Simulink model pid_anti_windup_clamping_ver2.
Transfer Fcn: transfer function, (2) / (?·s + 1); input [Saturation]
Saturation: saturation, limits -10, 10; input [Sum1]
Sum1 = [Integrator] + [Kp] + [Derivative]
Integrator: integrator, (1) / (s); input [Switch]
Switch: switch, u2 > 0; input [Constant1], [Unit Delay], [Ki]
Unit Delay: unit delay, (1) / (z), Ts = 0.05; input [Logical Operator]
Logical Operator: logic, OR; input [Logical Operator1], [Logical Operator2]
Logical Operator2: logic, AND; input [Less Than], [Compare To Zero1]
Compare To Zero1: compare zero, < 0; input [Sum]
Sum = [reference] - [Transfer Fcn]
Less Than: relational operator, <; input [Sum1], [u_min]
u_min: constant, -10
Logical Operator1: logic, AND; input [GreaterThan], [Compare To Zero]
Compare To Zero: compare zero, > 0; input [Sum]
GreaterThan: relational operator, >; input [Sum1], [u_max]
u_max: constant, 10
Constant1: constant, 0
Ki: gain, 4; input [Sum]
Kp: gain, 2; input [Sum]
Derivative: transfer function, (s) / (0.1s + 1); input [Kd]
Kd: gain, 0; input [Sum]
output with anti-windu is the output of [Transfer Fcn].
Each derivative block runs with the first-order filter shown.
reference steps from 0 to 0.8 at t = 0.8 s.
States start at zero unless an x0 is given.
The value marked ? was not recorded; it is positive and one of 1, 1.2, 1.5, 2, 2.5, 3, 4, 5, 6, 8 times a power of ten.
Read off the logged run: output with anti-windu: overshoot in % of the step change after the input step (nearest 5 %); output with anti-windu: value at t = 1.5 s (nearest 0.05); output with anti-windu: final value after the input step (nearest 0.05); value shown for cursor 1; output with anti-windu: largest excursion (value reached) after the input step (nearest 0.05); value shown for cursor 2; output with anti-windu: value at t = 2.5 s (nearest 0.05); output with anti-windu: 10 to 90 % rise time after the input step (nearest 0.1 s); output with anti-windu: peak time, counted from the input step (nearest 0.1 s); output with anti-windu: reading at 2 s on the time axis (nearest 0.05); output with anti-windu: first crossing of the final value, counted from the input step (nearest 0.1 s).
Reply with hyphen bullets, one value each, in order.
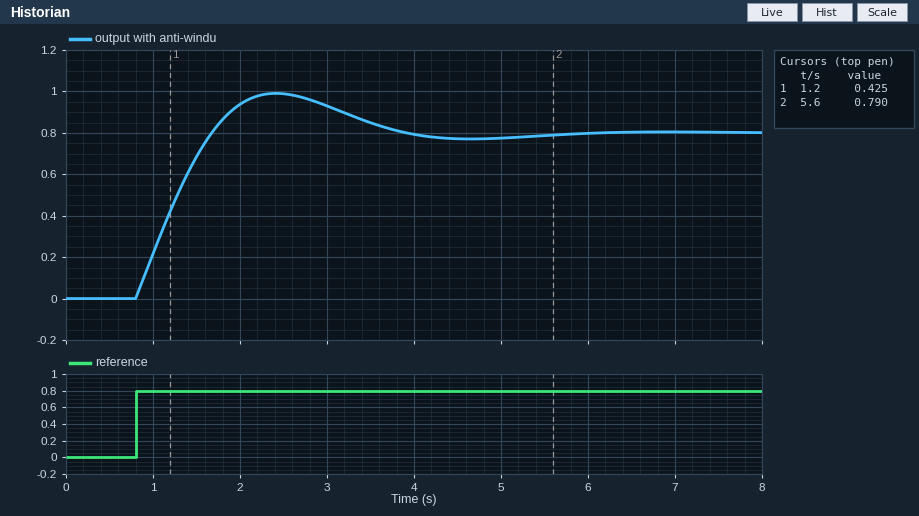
- 25 %
- 0.70
- 0.80
- 0.425
- 1.00
- 0.790
- 1.00
- 0.7 s
- 1.6 s
- 0.95
- 0.9 s
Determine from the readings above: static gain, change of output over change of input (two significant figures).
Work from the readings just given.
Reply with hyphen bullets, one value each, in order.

- 1.0
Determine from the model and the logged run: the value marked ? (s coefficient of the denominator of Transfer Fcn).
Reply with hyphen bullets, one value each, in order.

- 3
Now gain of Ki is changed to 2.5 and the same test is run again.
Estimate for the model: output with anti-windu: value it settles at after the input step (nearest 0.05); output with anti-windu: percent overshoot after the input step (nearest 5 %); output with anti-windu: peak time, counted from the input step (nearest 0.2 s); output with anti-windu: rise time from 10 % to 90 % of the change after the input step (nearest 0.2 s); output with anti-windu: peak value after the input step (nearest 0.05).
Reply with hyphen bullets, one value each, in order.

- 0.80
- 15 %
- 2.0 s
- 0.8 s
- 0.95
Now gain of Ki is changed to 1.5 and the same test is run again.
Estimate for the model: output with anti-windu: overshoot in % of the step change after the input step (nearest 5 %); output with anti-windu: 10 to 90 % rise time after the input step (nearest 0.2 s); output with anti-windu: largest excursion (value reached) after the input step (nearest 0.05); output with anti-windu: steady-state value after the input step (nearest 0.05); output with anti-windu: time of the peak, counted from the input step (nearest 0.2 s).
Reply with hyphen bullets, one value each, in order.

- 10 %
- 1.0 s
- 0.85
- 0.80
- 2.6 s
